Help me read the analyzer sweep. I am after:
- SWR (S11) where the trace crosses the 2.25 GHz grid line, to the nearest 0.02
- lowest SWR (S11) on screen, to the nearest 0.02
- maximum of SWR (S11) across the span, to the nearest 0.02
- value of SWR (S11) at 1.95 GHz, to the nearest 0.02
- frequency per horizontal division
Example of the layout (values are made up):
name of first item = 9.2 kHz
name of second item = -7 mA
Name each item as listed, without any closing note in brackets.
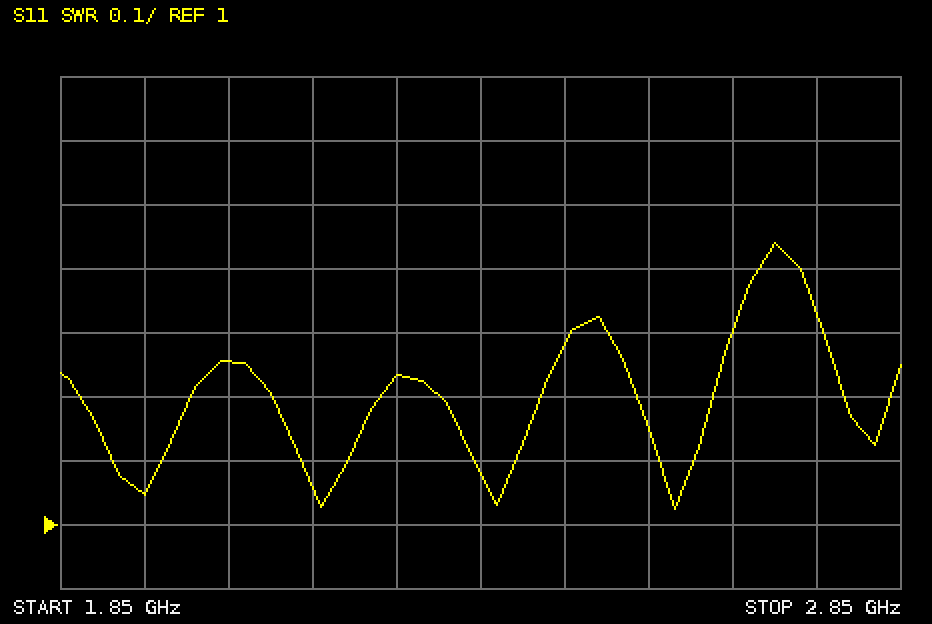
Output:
SWR (S11) where the trace crosses the 2.25 GHz grid line, to the nearest 0.02 = 1.24
lowest SWR (S11) on screen, to the nearest 0.02 = 1.02
maximum of SWR (S11) across the span, to the nearest 0.02 = 1.44
value of SWR (S11) at 1.95 GHz, to the nearest 0.02 = 1.04
frequency per horizontal division = 100 MHz
